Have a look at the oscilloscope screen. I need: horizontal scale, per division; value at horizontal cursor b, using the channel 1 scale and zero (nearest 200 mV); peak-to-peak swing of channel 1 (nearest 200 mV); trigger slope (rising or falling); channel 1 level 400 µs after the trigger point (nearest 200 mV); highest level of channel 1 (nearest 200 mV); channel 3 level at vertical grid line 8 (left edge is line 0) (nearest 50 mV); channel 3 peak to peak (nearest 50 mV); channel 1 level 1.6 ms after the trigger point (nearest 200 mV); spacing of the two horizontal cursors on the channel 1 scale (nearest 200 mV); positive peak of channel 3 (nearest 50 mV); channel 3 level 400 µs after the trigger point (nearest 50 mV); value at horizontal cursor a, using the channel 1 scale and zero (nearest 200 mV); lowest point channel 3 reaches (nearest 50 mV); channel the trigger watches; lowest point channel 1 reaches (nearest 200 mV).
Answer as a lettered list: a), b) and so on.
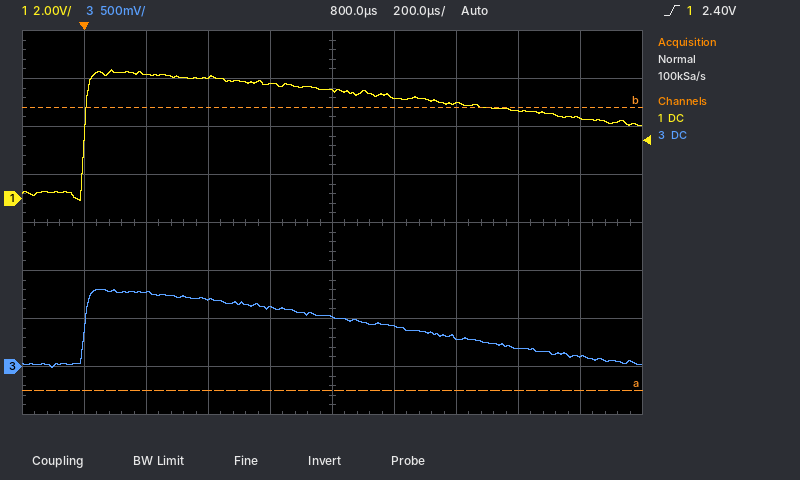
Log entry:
a) 200 µs
b) 3.8 V
c) 5.4 V
d) rising
e) 5.0 V
f) 5.4 V
g) 200 mV
h) 800 mV
i) 3.4 V
j) 11.8 V
k) 800 mV
l) 700 mV
m) -8.0 V
n) 0 mV
o) channel 1
p) 0.0 V
